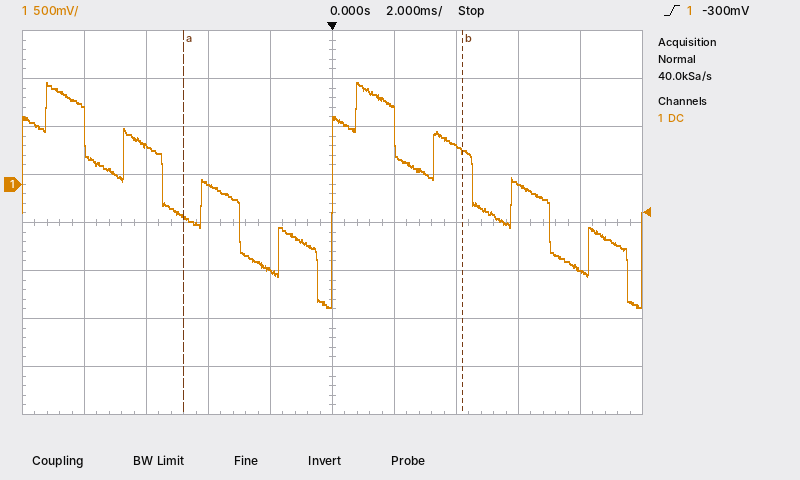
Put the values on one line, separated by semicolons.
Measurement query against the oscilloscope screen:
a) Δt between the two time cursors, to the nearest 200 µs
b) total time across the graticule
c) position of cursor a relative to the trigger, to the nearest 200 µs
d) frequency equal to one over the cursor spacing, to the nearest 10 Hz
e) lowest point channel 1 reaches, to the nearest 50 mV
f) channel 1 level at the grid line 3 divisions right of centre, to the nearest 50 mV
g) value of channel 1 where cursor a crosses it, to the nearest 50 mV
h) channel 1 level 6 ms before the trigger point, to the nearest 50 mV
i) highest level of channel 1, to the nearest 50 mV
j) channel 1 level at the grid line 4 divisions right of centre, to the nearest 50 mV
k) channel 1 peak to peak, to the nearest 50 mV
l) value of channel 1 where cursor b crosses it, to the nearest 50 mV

9.0 ms; 20 ms; -4.8 ms; 110 Hz; -1.30 V; 0 mV; -350 mV; 400 mV; 1.05 V; -900 mV; 2.35 V; 350 mV
